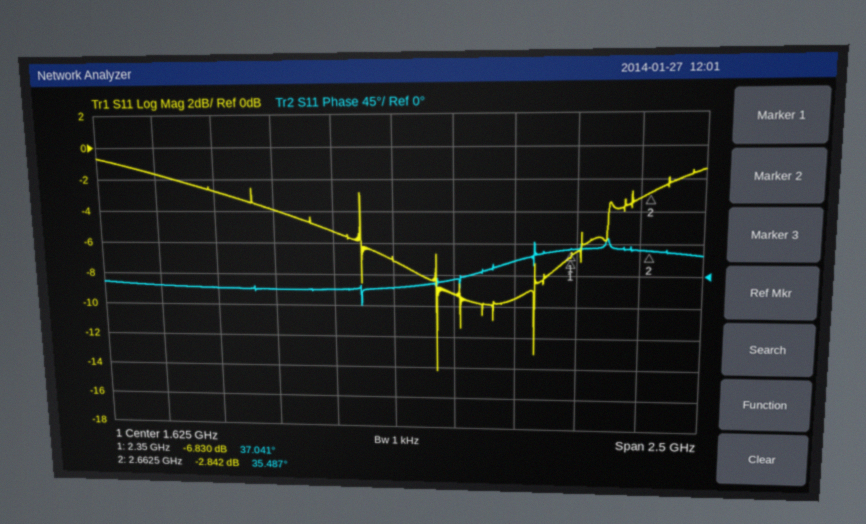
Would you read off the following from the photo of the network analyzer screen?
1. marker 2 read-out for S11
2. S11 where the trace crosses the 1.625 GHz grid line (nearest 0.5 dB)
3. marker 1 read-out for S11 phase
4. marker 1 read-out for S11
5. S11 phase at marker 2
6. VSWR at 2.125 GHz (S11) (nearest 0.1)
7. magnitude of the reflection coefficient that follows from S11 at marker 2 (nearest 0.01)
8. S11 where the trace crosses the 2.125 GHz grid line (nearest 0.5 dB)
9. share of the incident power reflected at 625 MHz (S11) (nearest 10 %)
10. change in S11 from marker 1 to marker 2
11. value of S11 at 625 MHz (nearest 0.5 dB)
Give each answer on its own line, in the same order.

-2.842 dB
-7.0 dB
37.041°
-6.830 dB
35.487°
2.0
0.72
-9.5 dB
70 %
3.988 dB
-1.5 dB
